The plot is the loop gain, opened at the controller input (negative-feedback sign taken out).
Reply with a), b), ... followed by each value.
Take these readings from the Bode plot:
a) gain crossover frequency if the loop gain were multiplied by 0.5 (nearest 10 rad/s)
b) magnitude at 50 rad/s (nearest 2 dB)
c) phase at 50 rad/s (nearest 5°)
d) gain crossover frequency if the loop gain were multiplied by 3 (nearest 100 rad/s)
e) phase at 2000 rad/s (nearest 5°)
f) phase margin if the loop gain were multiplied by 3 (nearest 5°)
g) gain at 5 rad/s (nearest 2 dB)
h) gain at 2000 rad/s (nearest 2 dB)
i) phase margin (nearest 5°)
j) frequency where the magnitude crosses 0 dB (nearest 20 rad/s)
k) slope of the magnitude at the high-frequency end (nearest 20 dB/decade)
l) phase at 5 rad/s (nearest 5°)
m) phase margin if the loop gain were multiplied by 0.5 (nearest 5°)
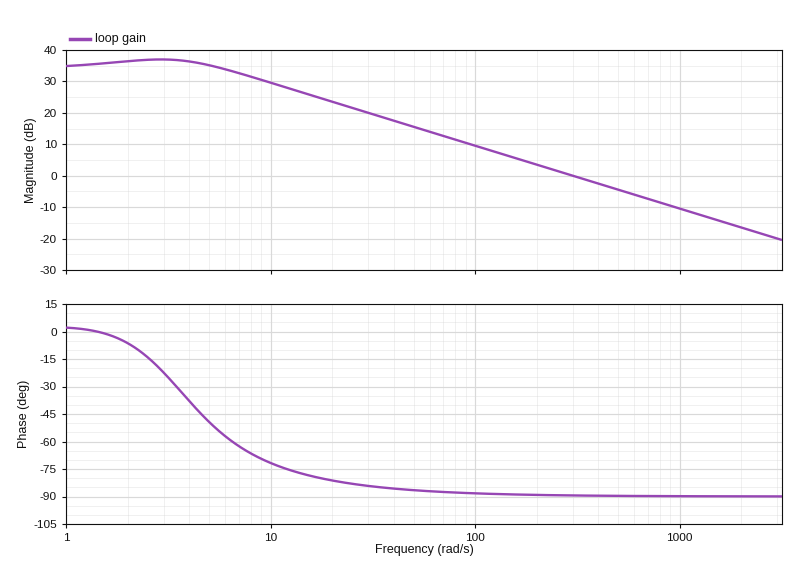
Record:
a) 150 rad/s
b) 16 dB
c) -85°
d) 900 rad/s
e) -90°
f) 90°
g) 36 dB
h) -16 dB
i) 90°
j) 300 rad/s
k) -20 dB/decade
l) -50°
m) 90°
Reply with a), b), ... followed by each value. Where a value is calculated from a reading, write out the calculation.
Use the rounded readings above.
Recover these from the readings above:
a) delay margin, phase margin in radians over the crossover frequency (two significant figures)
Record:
a) 90 × π / 180 / 300 = 0.0052 s
